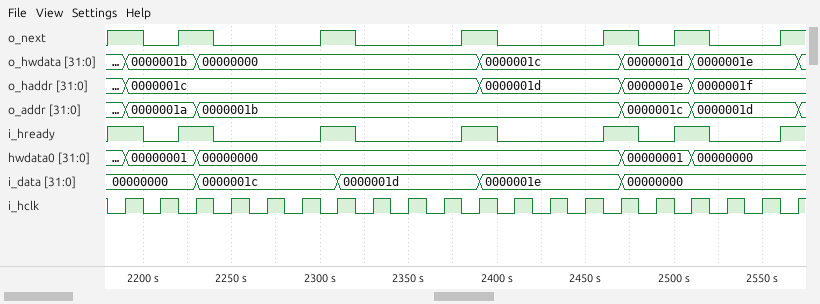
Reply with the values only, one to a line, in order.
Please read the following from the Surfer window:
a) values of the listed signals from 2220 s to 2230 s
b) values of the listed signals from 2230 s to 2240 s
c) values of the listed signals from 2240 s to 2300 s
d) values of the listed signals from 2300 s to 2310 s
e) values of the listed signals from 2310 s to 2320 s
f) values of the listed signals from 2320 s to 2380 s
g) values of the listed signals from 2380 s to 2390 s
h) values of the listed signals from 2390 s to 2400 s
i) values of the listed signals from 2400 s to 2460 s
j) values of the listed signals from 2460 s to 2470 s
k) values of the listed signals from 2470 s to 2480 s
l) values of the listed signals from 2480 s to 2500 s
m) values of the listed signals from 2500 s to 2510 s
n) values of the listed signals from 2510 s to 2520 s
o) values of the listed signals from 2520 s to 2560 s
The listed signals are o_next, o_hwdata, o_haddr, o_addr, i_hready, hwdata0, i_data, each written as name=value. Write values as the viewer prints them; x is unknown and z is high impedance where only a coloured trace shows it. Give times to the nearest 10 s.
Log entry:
o_next=1, o_hwdata=0000001b, o_haddr=0000001c, o_addr=0000001a, i_hready=1, hwdata0=00000001, i_data=00000000
o_next=1, o_hwdata=00000000, o_haddr=0000001c, o_addr=0000001b, i_hready=1, hwdata0=00000000, i_data=0000001c
o_next=0, o_hwdata=00000000, o_haddr=0000001c, o_addr=0000001b, i_hready=0, hwdata0=00000000, i_data=0000001c
o_next=1, o_hwdata=00000000, o_haddr=0000001c, o_addr=0000001b, i_hready=1, hwdata0=00000000, i_data=0000001c
o_next=1, o_hwdata=00000000, o_haddr=0000001c, o_addr=0000001b, i_hready=1, hwdata0=00000000, i_data=0000001d
o_next=0, o_hwdata=00000000, o_haddr=0000001c, o_addr=0000001b, i_hready=0, hwdata0=00000000, i_data=0000001d
o_next=1, o_hwdata=00000000, o_haddr=0000001c, o_addr=0000001b, i_hready=1, hwdata0=00000000, i_data=0000001d
o_next=1, o_hwdata=0000001c, o_haddr=0000001d, o_addr=0000001b, i_hready=1, hwdata0=00000000, i_data=0000001e
o_next=0, o_hwdata=0000001c, o_haddr=0000001d, o_addr=0000001b, i_hready=0, hwdata0=00000000, i_data=0000001e
o_next=1, o_hwdata=0000001c, o_haddr=0000001d, o_addr=0000001b, i_hready=1, hwdata0=00000000, i_data=0000001e
o_next=1, o_hwdata=0000001d, o_haddr=0000001e, o_addr=0000001c, i_hready=1, hwdata0=00000001, i_data=00000000
o_next=0, o_hwdata=0000001d, o_haddr=0000001e, o_addr=0000001c, i_hready=0, hwdata0=00000001, i_data=00000000
o_next=1, o_hwdata=0000001d, o_haddr=0000001e, o_addr=0000001c, i_hready=1, hwdata0=00000001, i_data=00000000
o_next=1, o_hwdata=0000001e, o_haddr=0000001f, o_addr=0000001d, i_hready=1, hwdata0=00000000, i_data=00000000
o_next=0, o_hwdata=0000001e, o_haddr=0000001f, o_addr=0000001d, i_hready=0, hwdata0=00000000, i_data=00000000
